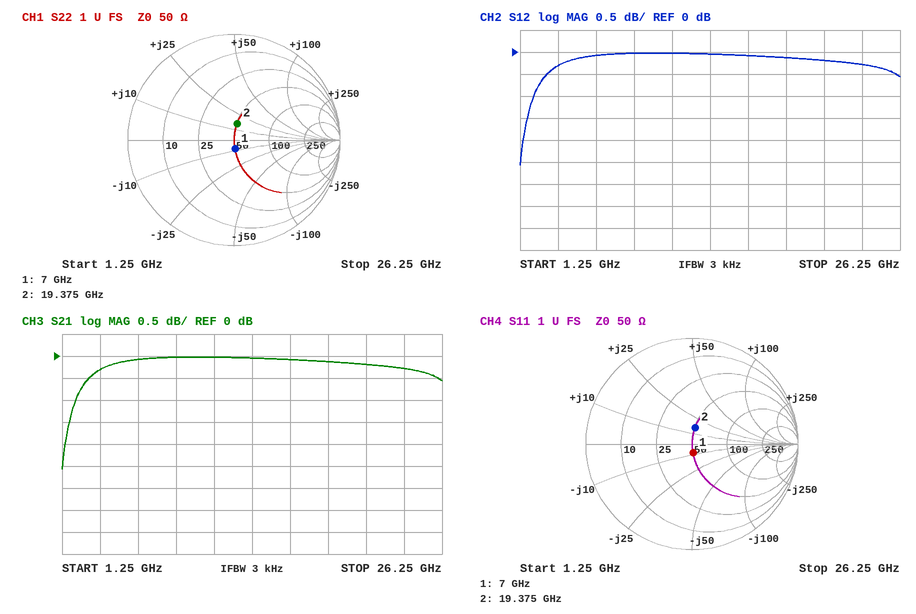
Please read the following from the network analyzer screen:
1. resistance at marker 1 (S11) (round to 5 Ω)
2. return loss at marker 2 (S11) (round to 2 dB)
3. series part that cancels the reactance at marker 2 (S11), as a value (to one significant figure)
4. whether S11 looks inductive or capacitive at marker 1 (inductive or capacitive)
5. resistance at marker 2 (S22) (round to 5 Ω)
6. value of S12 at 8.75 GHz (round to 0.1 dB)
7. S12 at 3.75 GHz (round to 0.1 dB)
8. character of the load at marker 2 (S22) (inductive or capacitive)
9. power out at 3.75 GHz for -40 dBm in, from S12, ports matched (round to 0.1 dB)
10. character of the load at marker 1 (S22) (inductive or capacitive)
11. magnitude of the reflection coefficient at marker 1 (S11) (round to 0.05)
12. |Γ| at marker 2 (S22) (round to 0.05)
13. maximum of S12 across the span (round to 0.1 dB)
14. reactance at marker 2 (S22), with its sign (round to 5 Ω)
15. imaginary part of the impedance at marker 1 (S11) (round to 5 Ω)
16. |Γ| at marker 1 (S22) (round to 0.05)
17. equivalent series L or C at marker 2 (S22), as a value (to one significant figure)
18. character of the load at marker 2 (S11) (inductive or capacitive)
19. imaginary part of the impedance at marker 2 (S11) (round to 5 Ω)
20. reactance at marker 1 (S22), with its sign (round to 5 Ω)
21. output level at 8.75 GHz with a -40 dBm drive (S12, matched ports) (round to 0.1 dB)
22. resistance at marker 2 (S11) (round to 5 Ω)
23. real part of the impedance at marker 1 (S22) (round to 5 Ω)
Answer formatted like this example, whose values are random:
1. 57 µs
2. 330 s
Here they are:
1. 50 Ω
2. 16 dB
3. 500 fF
4. capacitive
5. 50 Ω
6. 0.0 dB
7. -0.3 dB
8. inductive
9. -40.3 dBm
10. capacitive
11. 0.10
12. 0.15
13. 0.0 dB
14. +15 Ω
15. -10 Ω
16. 0.10
17. 100 pH
18. inductive
19. +15 Ω
20. -10 Ω
21. -40.0 dBm
22. 50 Ω
23. 50 Ω
